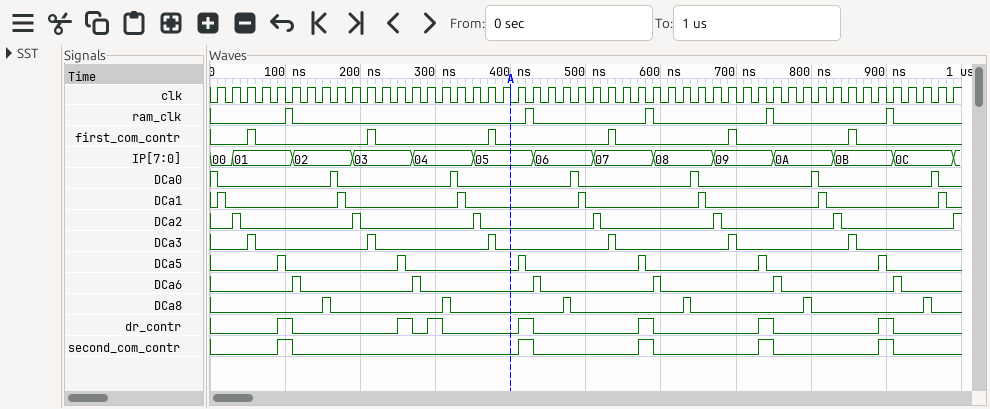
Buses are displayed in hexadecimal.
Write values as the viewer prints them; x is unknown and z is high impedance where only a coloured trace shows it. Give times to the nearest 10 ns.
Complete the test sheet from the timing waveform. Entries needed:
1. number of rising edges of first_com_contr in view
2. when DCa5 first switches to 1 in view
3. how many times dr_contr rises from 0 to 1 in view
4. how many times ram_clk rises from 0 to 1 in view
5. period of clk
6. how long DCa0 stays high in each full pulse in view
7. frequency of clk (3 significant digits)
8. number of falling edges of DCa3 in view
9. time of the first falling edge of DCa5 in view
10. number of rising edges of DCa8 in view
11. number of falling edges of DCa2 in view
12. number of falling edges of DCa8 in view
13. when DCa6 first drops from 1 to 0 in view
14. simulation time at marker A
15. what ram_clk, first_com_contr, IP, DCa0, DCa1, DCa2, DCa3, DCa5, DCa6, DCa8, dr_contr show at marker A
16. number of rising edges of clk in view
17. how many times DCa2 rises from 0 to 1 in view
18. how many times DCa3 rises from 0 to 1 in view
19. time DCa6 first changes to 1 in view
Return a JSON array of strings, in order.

["6", "90 ns", "7", "5", "20 ns", "10 ns, 10 ns, 10 ns, 10 ns, 10 ns, 10 ns", "50.0 MHz", "6", "100 ns", "6", "6", "6", "120 ns", "400 ns", "ram_clk=0, first_com_contr=0, IP=05, DCa0=0, DCa1=0, DCa2=0, DCa3=0, DCa5=0, DCa6=0, DCa8=0, dr_contr=0", "50", "7", "6", "110 ns"]
